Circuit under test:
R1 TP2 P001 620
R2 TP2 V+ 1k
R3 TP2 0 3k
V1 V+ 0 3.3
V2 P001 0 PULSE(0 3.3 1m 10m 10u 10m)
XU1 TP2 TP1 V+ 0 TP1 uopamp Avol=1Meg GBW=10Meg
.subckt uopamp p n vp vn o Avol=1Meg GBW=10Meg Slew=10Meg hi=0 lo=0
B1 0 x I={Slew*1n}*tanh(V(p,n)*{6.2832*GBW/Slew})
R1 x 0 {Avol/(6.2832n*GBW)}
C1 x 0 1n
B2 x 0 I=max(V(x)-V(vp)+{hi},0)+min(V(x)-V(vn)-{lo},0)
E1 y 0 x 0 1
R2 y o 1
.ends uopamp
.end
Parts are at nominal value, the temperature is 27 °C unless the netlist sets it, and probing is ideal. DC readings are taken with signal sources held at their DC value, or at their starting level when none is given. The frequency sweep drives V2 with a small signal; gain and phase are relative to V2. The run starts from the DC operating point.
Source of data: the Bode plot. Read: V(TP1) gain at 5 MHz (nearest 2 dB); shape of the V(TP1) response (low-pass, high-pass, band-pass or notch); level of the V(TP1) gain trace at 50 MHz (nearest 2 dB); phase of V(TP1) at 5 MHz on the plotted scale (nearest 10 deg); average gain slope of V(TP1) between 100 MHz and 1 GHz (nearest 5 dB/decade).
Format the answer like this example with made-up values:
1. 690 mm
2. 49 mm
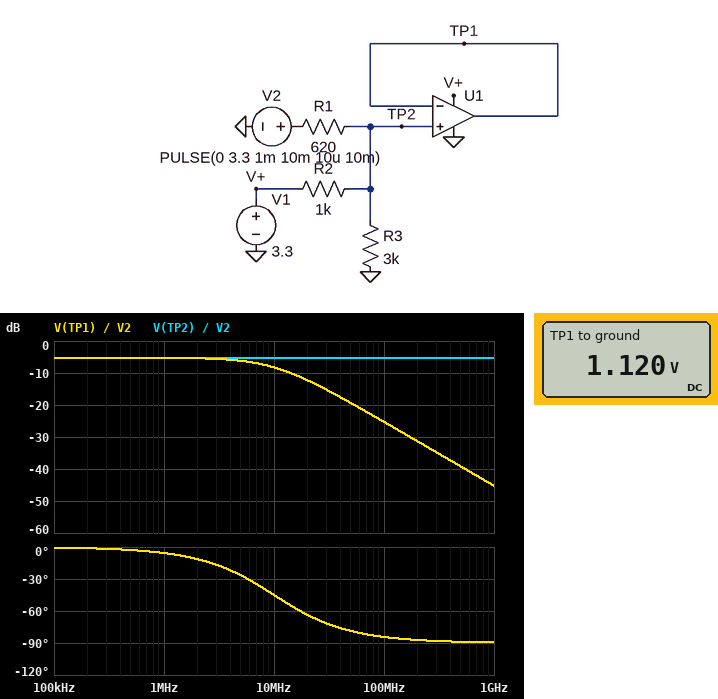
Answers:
1. -6 dB
2. low-pass
3. -20 dB
4. -30 deg
5. -20 dB/decade
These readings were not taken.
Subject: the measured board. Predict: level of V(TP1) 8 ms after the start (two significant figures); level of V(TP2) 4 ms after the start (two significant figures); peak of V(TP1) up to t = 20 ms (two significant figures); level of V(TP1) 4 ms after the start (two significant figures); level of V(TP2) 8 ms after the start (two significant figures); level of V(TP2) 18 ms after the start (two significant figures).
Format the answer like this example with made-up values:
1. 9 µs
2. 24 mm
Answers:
1. 2.4 V
2. 1.7 V
3. 2.9 V
4. 1.7 V
5. 2.4 V
6. 2.9 V
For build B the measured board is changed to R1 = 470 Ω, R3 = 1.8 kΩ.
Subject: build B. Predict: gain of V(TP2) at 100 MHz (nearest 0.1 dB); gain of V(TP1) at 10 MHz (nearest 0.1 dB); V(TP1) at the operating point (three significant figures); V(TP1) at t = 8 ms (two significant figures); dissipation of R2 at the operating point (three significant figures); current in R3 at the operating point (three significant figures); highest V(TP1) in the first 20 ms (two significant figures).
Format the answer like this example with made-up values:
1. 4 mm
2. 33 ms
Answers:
1. -4.8 dB
2. -7.8 dB
3. 896 mV
4. 2.2 V
5. 5.78 mW
6. 498 µA
7. 2.8 V
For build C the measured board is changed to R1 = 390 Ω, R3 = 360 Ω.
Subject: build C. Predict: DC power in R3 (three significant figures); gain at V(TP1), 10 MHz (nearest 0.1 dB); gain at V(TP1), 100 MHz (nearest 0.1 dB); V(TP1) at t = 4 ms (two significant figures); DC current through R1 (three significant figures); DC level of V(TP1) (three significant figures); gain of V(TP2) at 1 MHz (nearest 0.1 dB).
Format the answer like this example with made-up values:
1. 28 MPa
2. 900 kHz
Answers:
1. 752 µW
2. -10.9 dB
3. -27.9 dB
4. 920 mV
5. 1.33 mA
6. 520 mV
7. -7.9 dB
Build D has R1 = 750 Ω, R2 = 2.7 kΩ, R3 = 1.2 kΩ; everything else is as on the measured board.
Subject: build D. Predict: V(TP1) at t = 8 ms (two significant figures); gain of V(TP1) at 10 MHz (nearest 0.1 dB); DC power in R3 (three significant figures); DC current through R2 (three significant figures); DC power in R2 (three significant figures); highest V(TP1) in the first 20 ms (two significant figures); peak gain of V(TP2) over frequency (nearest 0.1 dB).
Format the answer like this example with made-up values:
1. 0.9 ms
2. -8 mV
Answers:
1. 1.7 V
2. -8.6 dB
3. 193 µW
4. 1.04 mA
5. 2.94 mW
6. 2.2 V
7. -5.6 dB
